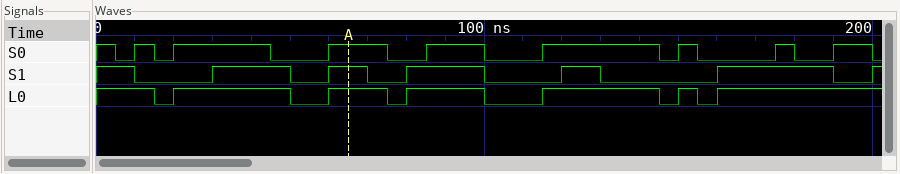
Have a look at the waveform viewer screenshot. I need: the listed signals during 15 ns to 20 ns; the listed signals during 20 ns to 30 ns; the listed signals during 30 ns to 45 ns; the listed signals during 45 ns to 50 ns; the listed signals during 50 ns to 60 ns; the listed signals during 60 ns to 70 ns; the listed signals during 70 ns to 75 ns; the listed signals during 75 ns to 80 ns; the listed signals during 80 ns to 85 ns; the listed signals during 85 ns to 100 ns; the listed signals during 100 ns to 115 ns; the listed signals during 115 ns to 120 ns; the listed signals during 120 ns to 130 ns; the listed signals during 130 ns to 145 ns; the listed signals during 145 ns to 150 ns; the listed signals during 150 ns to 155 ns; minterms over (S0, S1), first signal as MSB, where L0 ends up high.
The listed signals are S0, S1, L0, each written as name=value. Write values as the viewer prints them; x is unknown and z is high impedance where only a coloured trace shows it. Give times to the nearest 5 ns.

S0=0, S1=0, L0=0
S0=1, S1=0, L0=1
S0=1, S1=1, L0=1
S0=0, S1=1, L0=1
S0=0, S1=0, L0=0
S0=1, S1=1, L0=1
S0=1, S1=0, L0=1
S0=0, S1=0, L0=0
S0=0, S1=1, L0=1
S0=1, S1=1, L0=1
S0=0, S1=0, L0=0
S0=1, S1=0, L0=1
S0=1, S1=1, L0=1
S0=1, S1=0, L0=1
S0=0, S1=0, L0=0
S0=1, S1=0, L0=1
1, 2, 3
